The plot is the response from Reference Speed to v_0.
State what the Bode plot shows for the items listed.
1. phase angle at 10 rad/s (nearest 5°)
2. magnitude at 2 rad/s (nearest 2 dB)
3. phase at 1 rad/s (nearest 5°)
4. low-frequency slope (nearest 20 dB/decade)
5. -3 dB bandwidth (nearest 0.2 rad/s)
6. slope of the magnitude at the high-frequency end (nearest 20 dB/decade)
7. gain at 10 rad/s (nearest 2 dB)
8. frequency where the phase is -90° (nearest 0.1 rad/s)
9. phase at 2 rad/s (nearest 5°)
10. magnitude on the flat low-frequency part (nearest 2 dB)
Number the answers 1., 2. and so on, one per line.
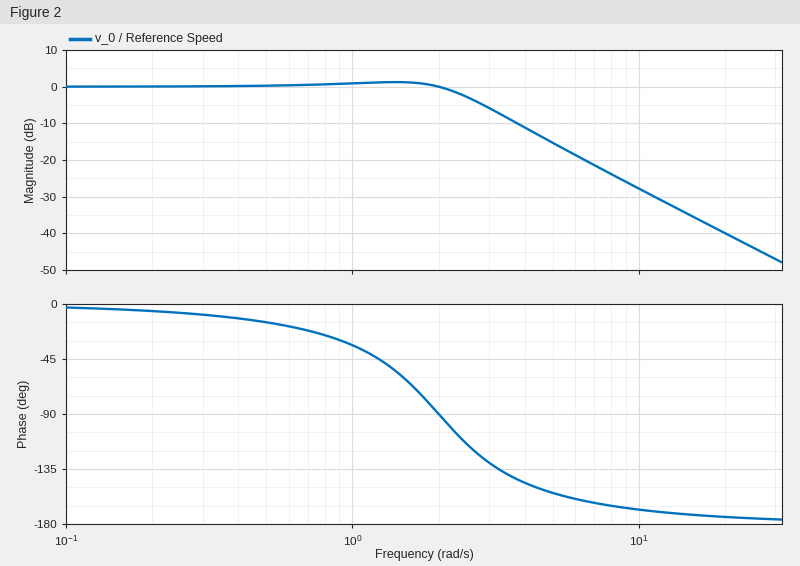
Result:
1. -170°
2. 0 dB
3. -35°
4. 0 dB/decade
5. 2.6 rad/s
6. -40 dB/decade
7. -28 dB
8. 2.0 rad/s
9. -90°
10. 0 dB
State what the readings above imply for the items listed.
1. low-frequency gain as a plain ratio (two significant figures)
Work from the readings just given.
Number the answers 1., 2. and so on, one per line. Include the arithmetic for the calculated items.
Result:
1. 10^(0 / 20) = 1.0
